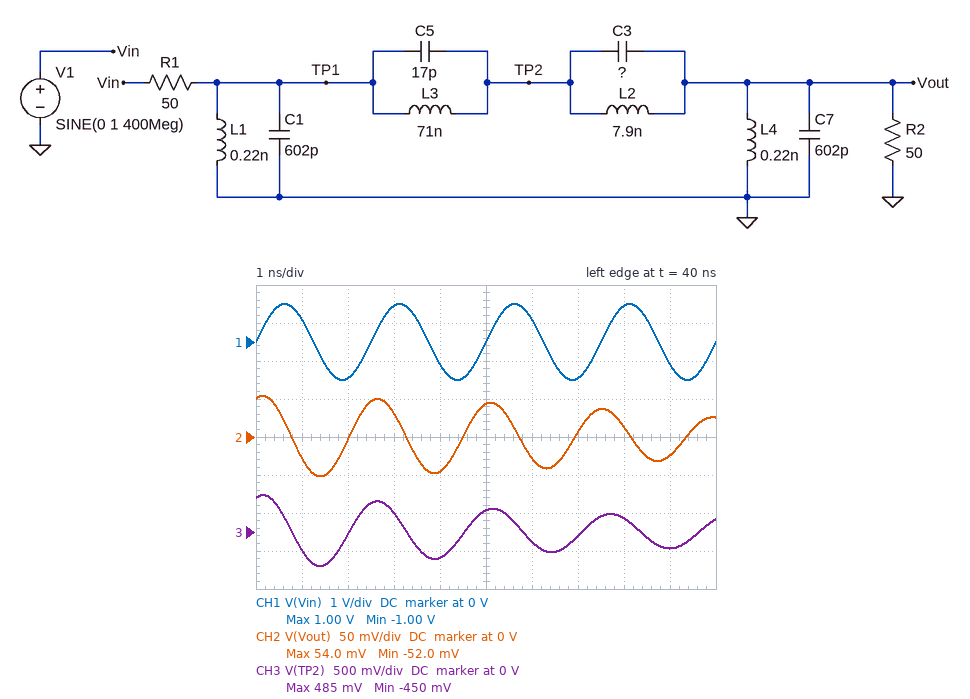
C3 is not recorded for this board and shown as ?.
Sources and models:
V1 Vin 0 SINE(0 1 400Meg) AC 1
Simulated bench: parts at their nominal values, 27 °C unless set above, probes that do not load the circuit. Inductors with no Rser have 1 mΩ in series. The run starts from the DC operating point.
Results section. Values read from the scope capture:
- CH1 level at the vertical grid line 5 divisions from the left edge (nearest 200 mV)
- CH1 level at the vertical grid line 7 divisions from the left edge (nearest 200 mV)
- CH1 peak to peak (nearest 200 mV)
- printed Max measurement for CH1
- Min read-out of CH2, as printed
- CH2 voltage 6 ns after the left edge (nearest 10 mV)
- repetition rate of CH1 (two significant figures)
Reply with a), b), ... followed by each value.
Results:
a) 0 V
b) -1.0 V
c) 2.0 V
d) 1.00 V
e) -52.0 mV
f) -30 mV
g) 400 MHz
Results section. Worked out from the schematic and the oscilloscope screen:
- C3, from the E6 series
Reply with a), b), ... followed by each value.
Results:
a) 4.7 pF
